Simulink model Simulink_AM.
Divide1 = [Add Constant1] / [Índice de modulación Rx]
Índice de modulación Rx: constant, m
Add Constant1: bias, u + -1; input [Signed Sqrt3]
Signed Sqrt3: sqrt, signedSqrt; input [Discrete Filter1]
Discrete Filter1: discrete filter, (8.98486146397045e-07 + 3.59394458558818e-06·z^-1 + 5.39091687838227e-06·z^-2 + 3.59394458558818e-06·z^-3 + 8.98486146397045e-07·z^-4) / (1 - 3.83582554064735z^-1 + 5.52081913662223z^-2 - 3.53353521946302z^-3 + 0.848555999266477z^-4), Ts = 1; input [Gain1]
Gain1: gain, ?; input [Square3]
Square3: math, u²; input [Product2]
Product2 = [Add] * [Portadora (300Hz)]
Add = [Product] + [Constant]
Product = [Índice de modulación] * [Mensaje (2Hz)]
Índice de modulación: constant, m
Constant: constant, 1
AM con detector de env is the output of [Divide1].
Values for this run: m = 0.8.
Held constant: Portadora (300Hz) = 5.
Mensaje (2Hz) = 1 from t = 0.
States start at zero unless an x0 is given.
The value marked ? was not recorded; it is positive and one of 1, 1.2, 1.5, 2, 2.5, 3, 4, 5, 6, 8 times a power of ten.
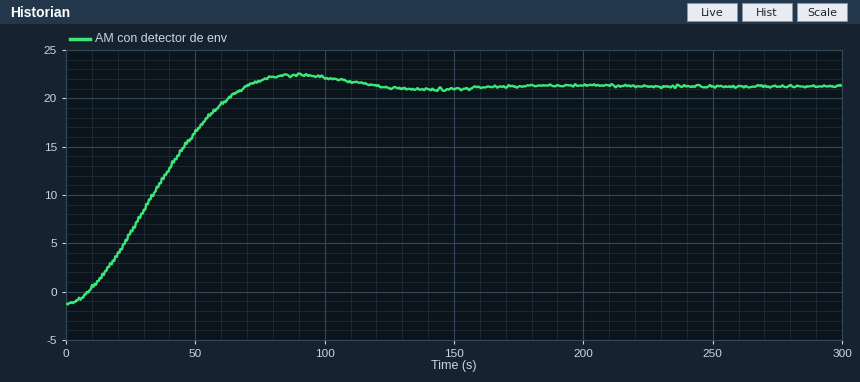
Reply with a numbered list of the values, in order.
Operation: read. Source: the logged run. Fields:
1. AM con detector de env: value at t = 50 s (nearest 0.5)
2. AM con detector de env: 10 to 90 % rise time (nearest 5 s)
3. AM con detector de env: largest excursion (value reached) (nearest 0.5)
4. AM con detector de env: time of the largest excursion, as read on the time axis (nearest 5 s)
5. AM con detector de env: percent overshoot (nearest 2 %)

1. 16.5
2. 45 s
3. 22.5
4. 90 s
5. 6 %
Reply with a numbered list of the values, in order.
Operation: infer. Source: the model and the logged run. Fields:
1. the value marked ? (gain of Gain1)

1. 4
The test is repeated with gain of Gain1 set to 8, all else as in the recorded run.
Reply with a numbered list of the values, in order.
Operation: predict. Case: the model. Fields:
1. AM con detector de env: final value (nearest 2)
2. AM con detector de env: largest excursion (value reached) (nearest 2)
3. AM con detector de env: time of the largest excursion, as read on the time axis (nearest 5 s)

1. 30
2. 32
3. 90 s
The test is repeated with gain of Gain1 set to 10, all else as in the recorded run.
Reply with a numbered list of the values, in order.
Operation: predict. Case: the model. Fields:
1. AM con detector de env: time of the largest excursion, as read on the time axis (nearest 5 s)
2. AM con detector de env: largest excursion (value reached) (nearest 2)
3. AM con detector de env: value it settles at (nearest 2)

1. 90 s
2. 36
3. 34
